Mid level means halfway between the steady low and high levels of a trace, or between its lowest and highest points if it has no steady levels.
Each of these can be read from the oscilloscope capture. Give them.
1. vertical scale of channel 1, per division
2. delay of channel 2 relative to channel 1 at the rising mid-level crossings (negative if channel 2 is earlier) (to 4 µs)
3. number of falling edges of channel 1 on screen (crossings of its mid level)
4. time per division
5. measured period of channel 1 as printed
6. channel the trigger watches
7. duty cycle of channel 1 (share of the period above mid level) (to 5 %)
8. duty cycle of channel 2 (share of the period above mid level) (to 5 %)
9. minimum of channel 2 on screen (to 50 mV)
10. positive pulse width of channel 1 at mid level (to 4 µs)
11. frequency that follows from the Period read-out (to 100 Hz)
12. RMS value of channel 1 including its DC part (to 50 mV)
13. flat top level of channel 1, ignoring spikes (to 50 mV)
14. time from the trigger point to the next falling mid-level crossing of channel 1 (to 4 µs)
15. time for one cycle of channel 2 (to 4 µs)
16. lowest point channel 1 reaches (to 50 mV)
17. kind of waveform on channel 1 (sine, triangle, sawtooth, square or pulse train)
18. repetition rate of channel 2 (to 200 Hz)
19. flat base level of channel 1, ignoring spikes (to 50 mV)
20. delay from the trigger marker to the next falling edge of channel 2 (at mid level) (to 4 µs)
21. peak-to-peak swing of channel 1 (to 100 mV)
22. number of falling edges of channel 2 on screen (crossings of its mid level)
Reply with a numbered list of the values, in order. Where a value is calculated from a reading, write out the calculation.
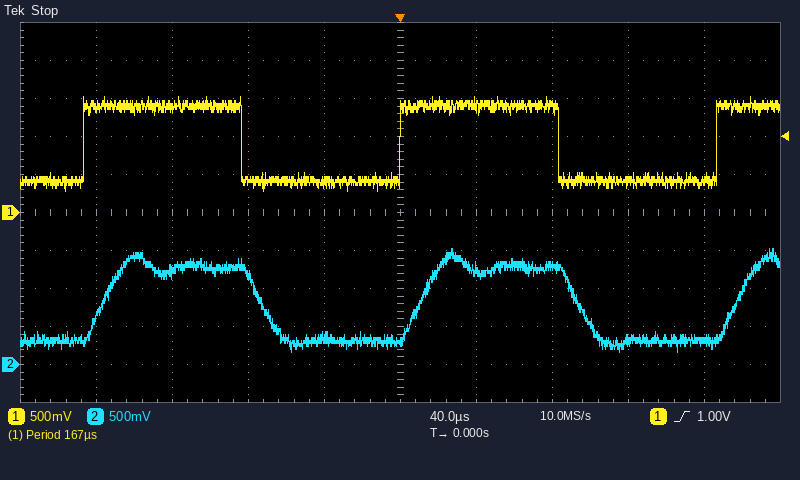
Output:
1. 500 mV
2. +12 µs
3. 2
4. 40 µs
5. 167 µs
6. channel 1
7. 50 %
8. 50 %
9. 150 mV
10. 84 µs
11. 1 / 167 µs ≈ 6.0 kHz
12. √(0.5 × (1.40 V)² + 0.5 × (400 mV)²) ≈ 1.03 V, so 1.05 V to the nearest 50 mV
13. 1.40 V
14. 84 µs
15. 168 µs
16. 300 mV
17. square
18. 1 / 168 µs ≈ 6.0 kHz
19. 400 mV
20. 92 µs
21. 1.20 V
22. 2
